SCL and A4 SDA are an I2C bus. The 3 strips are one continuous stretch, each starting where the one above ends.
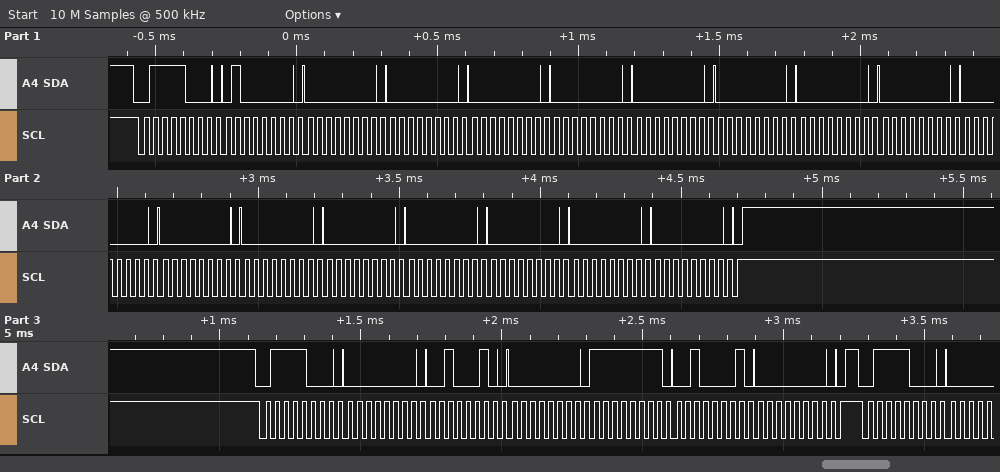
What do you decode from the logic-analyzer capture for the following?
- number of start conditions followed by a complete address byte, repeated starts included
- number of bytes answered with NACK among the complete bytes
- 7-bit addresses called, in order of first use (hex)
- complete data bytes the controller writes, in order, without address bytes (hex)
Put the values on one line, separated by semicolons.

3; 0; 0x3C; 40 00 00 00 00 00 00 00 00 00 00 00 00 00 00 00 00 00 22 00 FF 21 00
